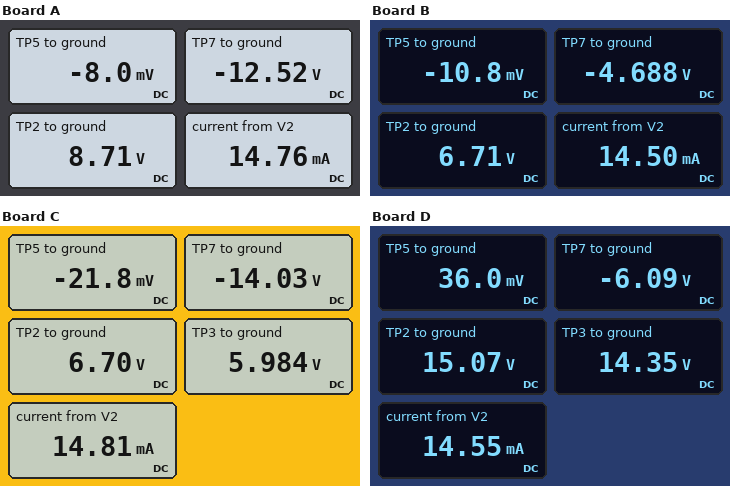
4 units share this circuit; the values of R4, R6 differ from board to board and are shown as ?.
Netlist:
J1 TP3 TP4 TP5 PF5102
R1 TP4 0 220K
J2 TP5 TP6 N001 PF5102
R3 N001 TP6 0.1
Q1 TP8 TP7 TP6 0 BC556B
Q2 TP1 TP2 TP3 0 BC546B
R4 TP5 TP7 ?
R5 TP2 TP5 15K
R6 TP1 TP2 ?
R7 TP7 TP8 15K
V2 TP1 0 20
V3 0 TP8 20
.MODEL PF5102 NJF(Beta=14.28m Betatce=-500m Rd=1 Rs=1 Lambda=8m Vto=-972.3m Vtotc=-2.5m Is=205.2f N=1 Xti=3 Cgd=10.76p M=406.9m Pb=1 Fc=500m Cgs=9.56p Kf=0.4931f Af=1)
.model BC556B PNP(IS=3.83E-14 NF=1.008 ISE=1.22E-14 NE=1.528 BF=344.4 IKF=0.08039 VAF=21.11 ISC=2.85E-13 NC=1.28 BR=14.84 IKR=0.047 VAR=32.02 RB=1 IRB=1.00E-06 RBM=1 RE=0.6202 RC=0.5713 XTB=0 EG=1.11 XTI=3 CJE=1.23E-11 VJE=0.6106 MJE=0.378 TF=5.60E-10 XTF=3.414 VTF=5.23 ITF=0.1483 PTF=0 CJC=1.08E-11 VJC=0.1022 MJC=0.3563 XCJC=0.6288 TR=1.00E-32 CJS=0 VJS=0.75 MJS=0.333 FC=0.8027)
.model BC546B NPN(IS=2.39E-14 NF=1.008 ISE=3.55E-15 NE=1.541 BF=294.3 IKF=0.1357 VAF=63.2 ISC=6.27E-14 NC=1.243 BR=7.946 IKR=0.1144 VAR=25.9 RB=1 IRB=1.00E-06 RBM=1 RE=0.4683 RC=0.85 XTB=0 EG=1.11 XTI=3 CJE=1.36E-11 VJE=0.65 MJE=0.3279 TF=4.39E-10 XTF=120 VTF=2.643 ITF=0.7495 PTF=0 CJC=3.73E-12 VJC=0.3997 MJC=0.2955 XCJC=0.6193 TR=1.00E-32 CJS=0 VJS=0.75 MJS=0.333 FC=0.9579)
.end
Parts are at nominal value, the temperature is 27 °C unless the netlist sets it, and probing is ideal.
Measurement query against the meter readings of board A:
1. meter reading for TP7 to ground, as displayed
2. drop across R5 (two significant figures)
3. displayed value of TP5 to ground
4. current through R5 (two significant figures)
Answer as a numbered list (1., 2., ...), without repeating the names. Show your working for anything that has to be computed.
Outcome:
1. -12.52 V
2. 8.71 V - (-8 mV) = 8.7 V
3. -8.0 mV
4. (8.71 V - (-8 mV)) / 15 kΩ = 580 µA
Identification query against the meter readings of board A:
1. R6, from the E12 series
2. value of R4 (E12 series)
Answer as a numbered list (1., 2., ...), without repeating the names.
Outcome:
1. 18 kΩ
2. 27 kΩ
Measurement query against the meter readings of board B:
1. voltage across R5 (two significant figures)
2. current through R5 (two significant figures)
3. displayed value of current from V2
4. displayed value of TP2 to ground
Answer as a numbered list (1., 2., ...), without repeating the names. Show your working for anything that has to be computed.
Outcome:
1. 6.71 V - (-10.8 mV) = 6.7 V
2. (6.71 V - (-10.8 mV)) / 15 kΩ = 450 µA
3. 14.50 mA
4. 6.71 V
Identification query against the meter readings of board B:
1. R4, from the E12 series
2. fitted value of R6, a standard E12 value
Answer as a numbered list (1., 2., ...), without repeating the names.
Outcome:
1. 4.7 kΩ
2. 27 kΩ
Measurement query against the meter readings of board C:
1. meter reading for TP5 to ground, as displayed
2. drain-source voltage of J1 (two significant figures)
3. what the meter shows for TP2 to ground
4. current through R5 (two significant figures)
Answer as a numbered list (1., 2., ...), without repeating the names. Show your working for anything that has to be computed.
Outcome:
1. -21.8 mV
2. 5.984 V - (-21.8 mV) = 6.0 V
3. 6.70 V
4. (6.7 V - (-21.8 mV)) / 15 kΩ = 450 µA
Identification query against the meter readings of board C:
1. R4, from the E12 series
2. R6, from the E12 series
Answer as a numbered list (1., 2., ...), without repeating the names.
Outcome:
1. 39 kΩ
2. 27 kΩ
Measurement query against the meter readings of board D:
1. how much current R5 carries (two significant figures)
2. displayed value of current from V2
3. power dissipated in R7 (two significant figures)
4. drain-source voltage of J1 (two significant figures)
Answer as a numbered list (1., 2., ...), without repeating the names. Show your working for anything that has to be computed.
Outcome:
1. (15.07 V - 36 mV) / 15 kΩ = 1.0 mA
2. 14.55 mA
3. (-6.09 V - (-20 V))^2 / 15 kΩ = 13 mW
4. 14.35 V - 36 mV = 14 V
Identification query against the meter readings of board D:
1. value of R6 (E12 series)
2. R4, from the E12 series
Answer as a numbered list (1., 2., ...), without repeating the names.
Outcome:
1. 4.7 kΩ
2. 6.8 kΩ
